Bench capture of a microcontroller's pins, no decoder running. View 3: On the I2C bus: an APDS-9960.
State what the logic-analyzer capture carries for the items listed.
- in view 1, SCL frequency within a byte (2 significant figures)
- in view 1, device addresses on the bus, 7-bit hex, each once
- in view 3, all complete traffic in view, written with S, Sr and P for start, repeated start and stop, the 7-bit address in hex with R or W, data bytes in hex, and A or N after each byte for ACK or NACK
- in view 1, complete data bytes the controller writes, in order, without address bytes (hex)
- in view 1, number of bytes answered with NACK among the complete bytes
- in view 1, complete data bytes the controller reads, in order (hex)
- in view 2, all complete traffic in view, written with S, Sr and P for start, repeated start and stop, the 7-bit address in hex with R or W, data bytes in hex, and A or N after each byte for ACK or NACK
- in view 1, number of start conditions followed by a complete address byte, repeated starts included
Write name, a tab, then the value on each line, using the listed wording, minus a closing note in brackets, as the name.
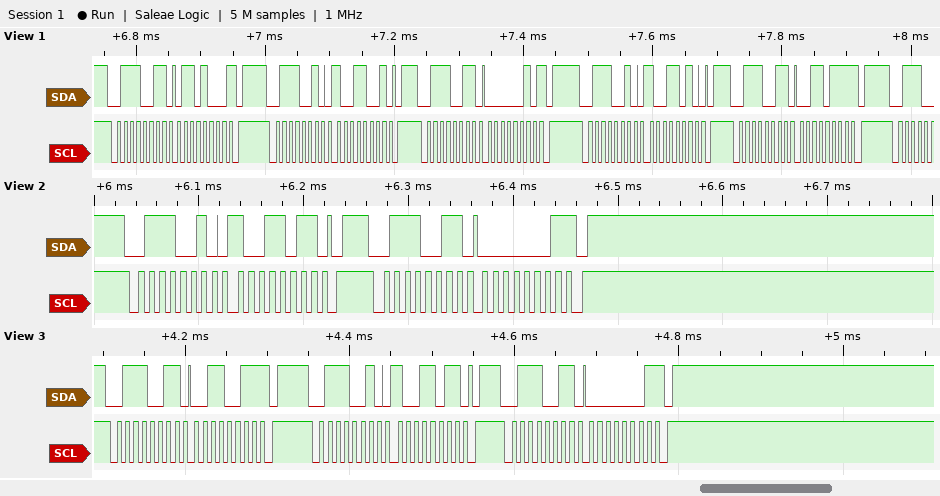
in view 1, SCL frequency within a byte	100 kHz
in view 1, device addresses on the bus, 7-bit hex, each once	0x39
in view 3, all complete traffic in view, written with S, Sr and P for start, repeated start and stop, the 7-bit address in hex with R or W, data bytes in hex, and A or N after each byte for ACK or NACK	S 39R A 33 N P S 39W A 9B A P S 39R A 01 N P
in view 1, complete data bytes the controller writes, in order, without address bytes	99 9A
in view 1, number of bytes answered with NACK among the complete bytes	3
in view 1, complete data bytes the controller reads, in order	68 02 37
in view 2, all complete traffic in view, written with S, Sr and P for start, repeated start and stop, the 7-bit address in hex with R or W, data bytes in hex, and A or N after each byte for ACK or NACK	S 39W A 9B A P S 39R A 01 N P
in view 1, number of start conditions followed by a complete address byte, repeated starts included	5
